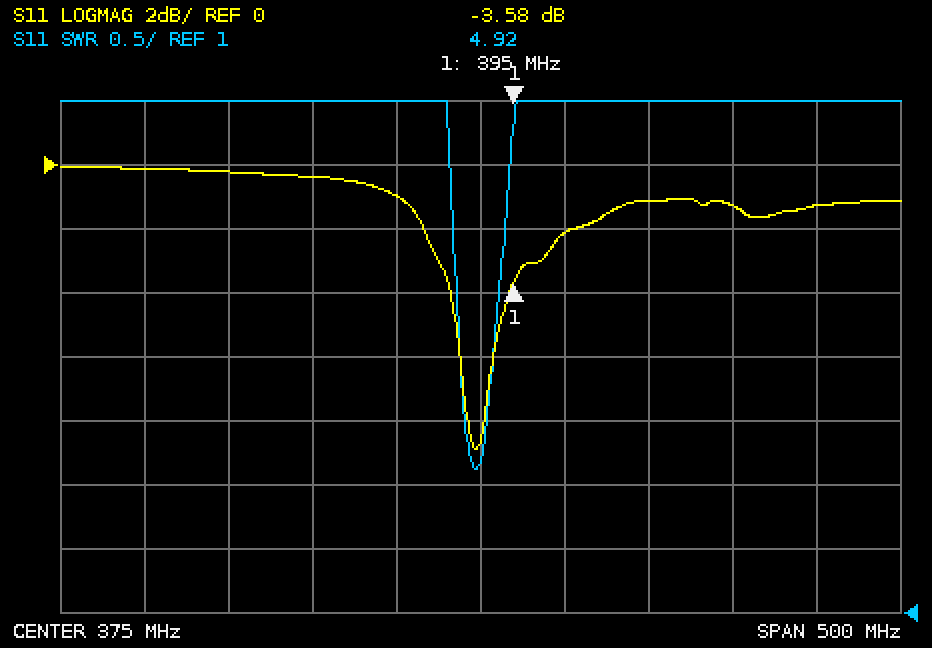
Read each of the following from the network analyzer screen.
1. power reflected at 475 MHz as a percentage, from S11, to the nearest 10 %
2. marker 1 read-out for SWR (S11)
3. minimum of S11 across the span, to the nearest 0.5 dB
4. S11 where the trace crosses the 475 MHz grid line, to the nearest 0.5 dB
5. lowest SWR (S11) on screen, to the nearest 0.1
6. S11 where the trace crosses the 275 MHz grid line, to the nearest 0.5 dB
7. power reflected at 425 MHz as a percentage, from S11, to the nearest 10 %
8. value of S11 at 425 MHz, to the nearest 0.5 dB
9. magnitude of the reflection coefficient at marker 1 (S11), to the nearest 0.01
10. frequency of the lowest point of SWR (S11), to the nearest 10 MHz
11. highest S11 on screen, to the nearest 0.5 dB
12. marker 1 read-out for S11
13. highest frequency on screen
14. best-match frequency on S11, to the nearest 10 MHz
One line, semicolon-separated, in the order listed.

80 %; 4.92; -9.0 dB; -1.0 dB; 2.1; -0.5 dB; 60 %; -2.0 dB; 0.66; 370 MHz; 0.0 dB; -3.58 dB; 625 MHz; 370 MHz
